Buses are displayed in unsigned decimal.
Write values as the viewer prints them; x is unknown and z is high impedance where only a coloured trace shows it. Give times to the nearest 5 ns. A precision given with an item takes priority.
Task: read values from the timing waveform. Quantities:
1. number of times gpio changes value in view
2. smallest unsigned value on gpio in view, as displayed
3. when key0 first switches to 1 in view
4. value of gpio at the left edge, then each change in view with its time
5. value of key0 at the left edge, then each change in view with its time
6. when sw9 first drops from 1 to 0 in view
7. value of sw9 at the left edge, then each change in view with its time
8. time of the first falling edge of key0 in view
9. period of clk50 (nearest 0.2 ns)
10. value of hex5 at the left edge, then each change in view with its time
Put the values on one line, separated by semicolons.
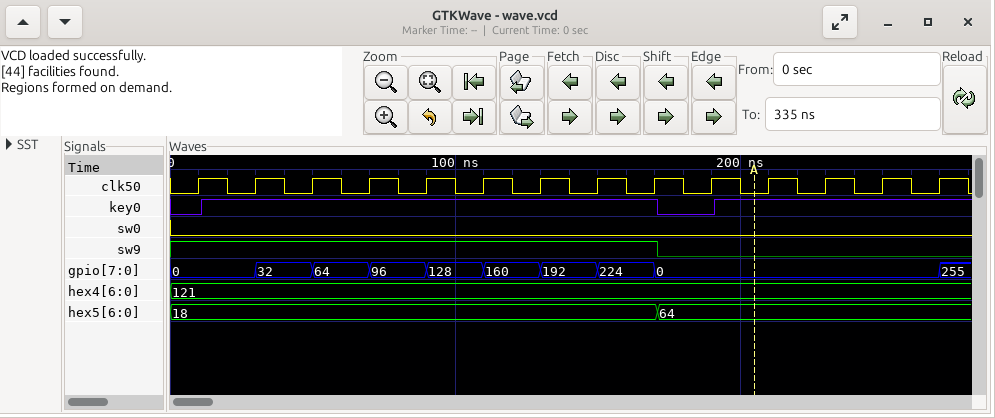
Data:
9; 0; 10 ns; 0, 32 at 30 ns, 64 at 50 ns, 96 at 70 ns, 128 at 90 ns, 160 at 110 ns, 192 at 130 ns, 224 at 150 ns, 0 at 170 ns, 255 at 270 ns; 0, 1 at 10 ns, 0 at 170 ns, 1 at 190 ns; 170 ns; 1, 0 at 170 ns; 170 ns; 20 ns; 18, 64 at 170 ns
